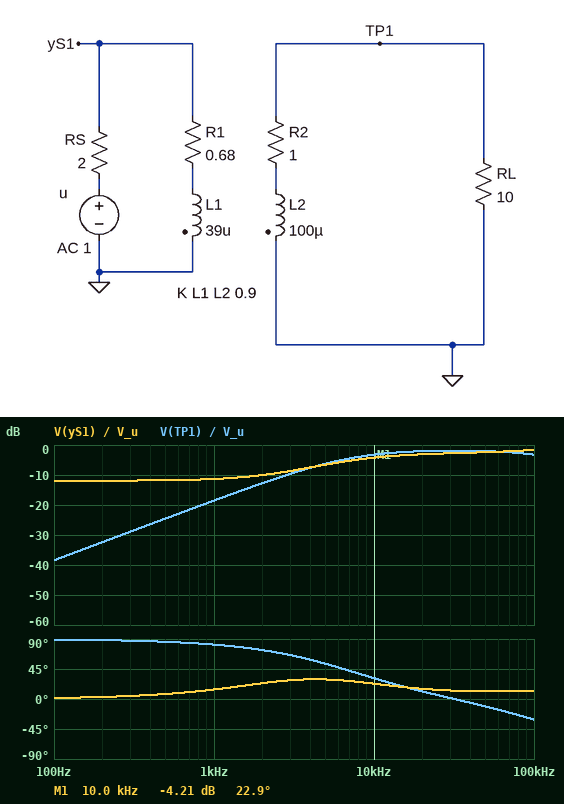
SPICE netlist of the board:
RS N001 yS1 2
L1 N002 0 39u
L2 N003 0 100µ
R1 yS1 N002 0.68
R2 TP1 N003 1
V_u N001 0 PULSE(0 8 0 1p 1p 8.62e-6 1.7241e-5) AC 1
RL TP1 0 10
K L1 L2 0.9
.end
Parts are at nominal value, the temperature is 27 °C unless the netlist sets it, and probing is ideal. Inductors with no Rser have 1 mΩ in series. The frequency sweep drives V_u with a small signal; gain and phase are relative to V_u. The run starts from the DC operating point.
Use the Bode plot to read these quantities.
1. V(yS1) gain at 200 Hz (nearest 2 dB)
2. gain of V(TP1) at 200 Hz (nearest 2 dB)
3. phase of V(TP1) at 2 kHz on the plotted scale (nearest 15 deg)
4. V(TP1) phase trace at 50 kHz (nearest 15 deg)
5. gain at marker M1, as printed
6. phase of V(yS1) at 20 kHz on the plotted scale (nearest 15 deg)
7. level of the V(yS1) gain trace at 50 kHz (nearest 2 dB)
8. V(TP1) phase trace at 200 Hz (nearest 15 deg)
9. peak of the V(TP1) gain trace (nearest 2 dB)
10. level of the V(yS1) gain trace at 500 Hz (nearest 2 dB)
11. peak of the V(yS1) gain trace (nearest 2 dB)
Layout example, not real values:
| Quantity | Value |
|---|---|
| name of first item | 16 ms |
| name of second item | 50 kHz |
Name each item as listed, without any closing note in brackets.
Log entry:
| Quantity | Value |
|---|---|
| V(yS1) gain at 200 Hz | -12 dB |
| gain of V(TP1) at 200 Hz | -32 dB |
| phase of V(TP1) at 2 kHz on the plotted scale | 75 deg |
| V(TP1) phase trace at 50 kHz | -15 deg |
| gain at marker M1, as printed | -4.21 dB |
| phase of V(yS1) at 20 kHz on the plotted scale | 15 deg |
| level of the V(yS1) gain trace at 50 kHz | -2 dB |
| V(TP1) phase trace at 200 Hz | 90 deg |
| peak of the V(TP1) gain trace | -2 dB |
| level of the V(yS1) gain trace at 500 Hz | -12 dB |
| peak of the V(yS1) gain trace | -2 dB |
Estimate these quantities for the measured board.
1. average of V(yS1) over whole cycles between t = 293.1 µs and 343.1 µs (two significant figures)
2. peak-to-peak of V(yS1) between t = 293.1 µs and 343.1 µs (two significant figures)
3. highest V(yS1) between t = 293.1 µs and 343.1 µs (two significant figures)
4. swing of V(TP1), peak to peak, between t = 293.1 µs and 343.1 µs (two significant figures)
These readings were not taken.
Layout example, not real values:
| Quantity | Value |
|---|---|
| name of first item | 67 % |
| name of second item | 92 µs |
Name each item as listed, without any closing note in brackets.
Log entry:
| Quantity | Value |
|---|---|
| average of V(yS1) over whole cycles between t = 293.1 µs and 343.1 µs | 1.0 V |
| peak-to-peak of V(yS1) between t = 293.1 µs and 343.1 µs | 11 V |
| highest V(yS1) between t = 293.1 µs and 343.1 µs | 6.5 V |
| swing of V(TP1), peak to peak, between t = 293.1 µs and 343.1 µs | 6.7 V |
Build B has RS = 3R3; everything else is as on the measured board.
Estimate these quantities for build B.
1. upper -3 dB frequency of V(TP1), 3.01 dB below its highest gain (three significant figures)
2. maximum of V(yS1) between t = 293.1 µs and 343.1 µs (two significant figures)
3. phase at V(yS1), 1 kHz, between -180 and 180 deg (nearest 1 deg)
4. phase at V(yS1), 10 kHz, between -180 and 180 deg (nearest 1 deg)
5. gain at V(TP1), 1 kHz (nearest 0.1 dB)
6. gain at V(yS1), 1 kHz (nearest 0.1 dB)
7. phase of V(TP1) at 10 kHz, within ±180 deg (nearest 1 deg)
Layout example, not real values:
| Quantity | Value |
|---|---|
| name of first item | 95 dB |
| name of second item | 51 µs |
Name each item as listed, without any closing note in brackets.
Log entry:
| Quantity | Value |
|---|---|
| upper -3 dB frequency of V(TP1), 3.01 dB below its highest gain | 186 kHz |
| maximum of V(yS1) between t = 293.1 µs and 343.1 µs | 6.7 V |
| phase at V(yS1), 1 kHz, between -180 and 180 deg | 16 deg |
| phase at V(yS1), 10 kHz, between -180 and 180 deg | 30 deg |
| gain at V(TP1), 1 kHz | -21.9 dB |
| gain at V(yS1), 1 kHz | -14.7 dB |
| phase of V(TP1) at 10 kHz, within ±180 deg | 38 deg |
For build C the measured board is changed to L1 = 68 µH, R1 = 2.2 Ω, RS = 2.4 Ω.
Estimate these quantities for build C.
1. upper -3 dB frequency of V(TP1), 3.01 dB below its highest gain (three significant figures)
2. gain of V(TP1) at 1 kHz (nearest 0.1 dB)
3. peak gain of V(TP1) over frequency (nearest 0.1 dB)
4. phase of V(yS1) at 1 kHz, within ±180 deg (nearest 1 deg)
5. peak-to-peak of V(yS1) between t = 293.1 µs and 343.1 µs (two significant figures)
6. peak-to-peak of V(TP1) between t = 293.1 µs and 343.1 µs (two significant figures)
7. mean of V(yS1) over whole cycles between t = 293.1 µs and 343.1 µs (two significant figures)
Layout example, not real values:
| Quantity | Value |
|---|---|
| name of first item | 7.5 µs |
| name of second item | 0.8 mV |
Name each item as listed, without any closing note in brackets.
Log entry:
| Quantity | Value |
|---|---|
| upper -3 dB frequency of V(TP1), 3.01 dB below its highest gain | 155 kHz |
| gain of V(TP1) at 1 kHz | -20.8 dB |
| peak gain of V(TP1) over frequency | -4.2 dB |
| phase of V(yS1) at 1 kHz, within ±180 deg | 6 deg |
| peak-to-peak of V(yS1) between t = 293.1 µs and 343.1 µs | 10 V |
| peak-to-peak of V(TP1) between t = 293.1 µs and 343.1 µs | 5.1 V |
| mean of V(yS1) over whole cycles between t = 293.1 µs and 343.1 µs | 1.9 V |
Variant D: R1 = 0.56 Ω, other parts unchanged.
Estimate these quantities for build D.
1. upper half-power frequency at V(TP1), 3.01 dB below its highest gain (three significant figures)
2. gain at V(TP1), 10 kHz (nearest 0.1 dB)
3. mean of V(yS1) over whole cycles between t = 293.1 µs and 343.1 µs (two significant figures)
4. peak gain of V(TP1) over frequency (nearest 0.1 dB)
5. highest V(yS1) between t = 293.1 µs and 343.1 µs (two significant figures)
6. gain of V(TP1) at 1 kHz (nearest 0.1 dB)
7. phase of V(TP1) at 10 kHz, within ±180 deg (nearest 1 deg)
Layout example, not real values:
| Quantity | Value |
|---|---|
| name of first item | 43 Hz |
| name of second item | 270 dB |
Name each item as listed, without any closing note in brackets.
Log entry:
| Quantity | Value |
|---|---|
| upper half-power frequency at V(TP1), 3.01 dB below its highest gain | 153 kHz |
| gain at V(TP1), 10 kHz | -3.0 dB |
| mean of V(yS1) over whole cycles between t = 293.1 µs and 343.1 µs | 880 mV |
| peak gain of V(TP1) over frequency | -1.7 dB |
| highest V(yS1) between t = 293.1 µs and 343.1 µs | 6.4 V |
| gain of V(TP1) at 1 kHz | -18.1 dB |
| phase of V(TP1) at 10 kHz, within ±180 deg | 30 deg |
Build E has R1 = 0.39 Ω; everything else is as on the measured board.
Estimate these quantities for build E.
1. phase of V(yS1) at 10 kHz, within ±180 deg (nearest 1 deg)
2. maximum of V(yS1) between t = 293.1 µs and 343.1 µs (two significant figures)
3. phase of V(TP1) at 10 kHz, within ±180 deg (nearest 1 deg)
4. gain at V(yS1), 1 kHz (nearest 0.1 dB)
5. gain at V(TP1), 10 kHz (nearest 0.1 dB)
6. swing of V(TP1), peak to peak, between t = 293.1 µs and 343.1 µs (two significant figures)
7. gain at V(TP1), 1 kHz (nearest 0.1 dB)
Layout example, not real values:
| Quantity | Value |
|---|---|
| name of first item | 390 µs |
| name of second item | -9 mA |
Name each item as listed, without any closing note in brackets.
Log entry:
| Quantity | Value |
|---|---|
| phase of V(yS1) at 10 kHz, within ±180 deg | 26 deg |
| maximum of V(yS1) between t = 293.1 µs and 343.1 µs | 6.2 V |
| phase of V(TP1) at 10 kHz, within ±180 deg | 29 deg |
| gain at V(yS1), 1 kHz | -14.2 dB |
| gain at V(TP1), 10 kHz | -2.7 dB |
| swing of V(TP1), peak to peak, between t = 293.1 µs and 343.1 µs | 6.9 V |
| gain at V(TP1), 1 kHz | -17.5 dB |
